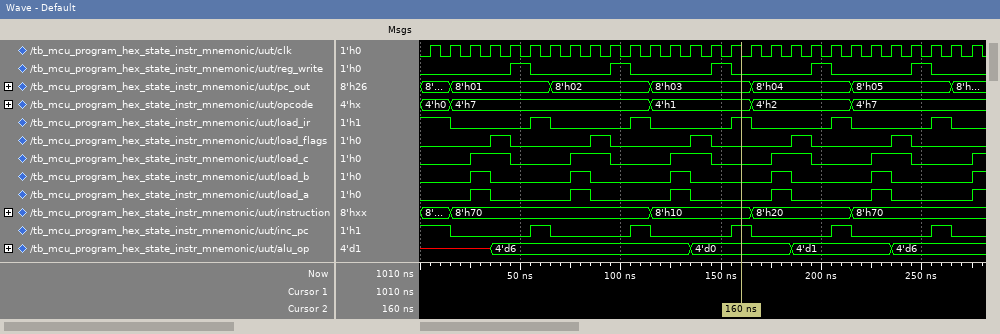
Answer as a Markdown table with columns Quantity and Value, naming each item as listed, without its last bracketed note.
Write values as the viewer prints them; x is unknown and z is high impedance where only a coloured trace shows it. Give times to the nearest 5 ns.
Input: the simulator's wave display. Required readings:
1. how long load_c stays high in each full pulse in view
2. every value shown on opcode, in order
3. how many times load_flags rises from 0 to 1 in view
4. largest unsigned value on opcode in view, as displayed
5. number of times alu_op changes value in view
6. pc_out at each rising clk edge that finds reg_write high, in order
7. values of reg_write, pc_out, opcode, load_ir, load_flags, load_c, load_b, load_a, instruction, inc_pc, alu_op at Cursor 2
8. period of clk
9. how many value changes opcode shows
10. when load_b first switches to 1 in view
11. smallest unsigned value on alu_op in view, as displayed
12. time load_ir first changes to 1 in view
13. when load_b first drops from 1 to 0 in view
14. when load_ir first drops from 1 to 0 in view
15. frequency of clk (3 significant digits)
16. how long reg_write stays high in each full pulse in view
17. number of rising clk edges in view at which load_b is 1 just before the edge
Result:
| Quantity | Value |
|---|---|
| how long load_c stays high in each full pulse in view | 20 ns, 20 ns, 20 ns, 20 ns, 20 ns |
| every value shown on opcode, in order | 4'h0, 4'h7, 4'h1, 4'h2, 4'h7 |
| how many times load_flags rises from 0 to 1 in view | 5 |
| largest unsigned value on opcode in view, as displayed | 4'h7 |
| number of times alu_op changes value in view | 4 |
| pc_out at each rising clk edge that finds reg_write high, in order | 8'h01, 8'h02, 8'h03, 8'h04, 8'h05 |
| values of reg_write, pc_out, opcode, load_ir, load_flags, load_c, load_b, load_a, instruction, inc_pc, alu_op at Cursor 2 | reg_write=0, pc_out=8'h03, opcode=4'h1, load_ir=1, load_flags=0, load_c=0, load_b=0, load_a=0, instruction=8'h10, inc_pc=1, alu_op=4'd0 |
| period of clk | 10 ns |
| how many value changes opcode shows | 4 |
| when load_b first switches to 1 in view | 25 ns |
| smallest unsigned value on alu_op in view, as displayed | 4'd0 |
| time load_ir first changes to 1 in view | 55 ns |
| when load_b first drops from 1 to 0 in view | 35 ns |
| when load_ir first drops from 1 to 0 in view | 15 ns |
| frequency of clk | 100 MHz |
| how long reg_write stays high in each full pulse in view | 10 ns, 10 ns, 10 ns, 10 ns, 10 ns |
| number of rising clk edges in view at which load_b is 1 just before the edge | 5 |
